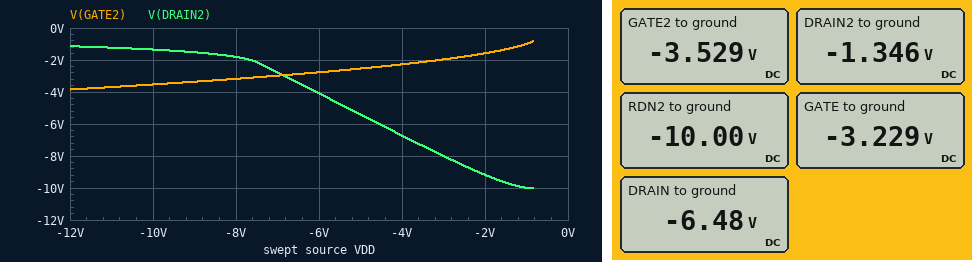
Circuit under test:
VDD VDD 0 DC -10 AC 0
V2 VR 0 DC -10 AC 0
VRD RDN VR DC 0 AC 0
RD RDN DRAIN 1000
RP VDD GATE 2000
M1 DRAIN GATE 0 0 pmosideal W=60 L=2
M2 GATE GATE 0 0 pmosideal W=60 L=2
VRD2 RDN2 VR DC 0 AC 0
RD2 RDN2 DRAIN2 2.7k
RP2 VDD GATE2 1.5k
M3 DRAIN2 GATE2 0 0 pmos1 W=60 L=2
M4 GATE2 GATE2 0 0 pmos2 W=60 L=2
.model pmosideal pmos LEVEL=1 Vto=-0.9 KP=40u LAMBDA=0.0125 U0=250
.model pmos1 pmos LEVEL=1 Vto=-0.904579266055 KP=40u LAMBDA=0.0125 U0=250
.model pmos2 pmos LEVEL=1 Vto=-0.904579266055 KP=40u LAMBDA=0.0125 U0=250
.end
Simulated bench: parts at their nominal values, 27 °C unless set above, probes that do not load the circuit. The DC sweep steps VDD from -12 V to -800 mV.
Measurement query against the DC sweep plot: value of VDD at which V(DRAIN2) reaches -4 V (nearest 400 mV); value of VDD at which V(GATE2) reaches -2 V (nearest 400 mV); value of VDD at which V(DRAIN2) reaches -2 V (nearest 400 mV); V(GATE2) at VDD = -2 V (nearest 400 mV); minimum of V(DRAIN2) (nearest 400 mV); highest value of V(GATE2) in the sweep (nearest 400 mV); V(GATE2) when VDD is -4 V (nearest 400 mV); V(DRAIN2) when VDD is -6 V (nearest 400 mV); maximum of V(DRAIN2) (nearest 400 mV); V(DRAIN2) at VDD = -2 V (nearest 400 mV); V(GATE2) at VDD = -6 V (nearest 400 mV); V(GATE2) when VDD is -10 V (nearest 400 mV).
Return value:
-6.0 V
-3.2 V
-7.6 V
-1.6 V
-10.0 V
-800 mV
-2.4 V
-4.0 V
-1.2 V
-9.2 V
-2.8 V
-3.6 V
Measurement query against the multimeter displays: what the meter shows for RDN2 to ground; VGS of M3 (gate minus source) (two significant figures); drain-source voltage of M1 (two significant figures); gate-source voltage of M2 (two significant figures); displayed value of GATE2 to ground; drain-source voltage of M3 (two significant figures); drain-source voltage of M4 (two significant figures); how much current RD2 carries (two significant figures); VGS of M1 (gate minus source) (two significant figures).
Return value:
-10.00 V
-3.5 V
-6.5 V
-3.2 V
-3.529 V
-1.3 V
-3.5 V
3.2 mA
-3.2 V
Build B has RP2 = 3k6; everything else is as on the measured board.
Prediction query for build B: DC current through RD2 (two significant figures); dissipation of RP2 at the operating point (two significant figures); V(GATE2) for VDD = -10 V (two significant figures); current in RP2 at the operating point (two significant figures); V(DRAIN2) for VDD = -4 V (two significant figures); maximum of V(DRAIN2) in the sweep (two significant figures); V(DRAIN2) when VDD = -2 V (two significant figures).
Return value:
2.1 mA
15 mW
-2.7 V
2.0 mA
-8.3 V
-3.2 V
-9.5 V
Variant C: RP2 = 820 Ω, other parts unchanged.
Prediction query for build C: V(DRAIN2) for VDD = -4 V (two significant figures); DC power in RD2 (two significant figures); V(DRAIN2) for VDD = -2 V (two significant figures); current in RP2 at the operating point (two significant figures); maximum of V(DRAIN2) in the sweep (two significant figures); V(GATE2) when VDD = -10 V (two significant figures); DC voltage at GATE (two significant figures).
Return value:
-5.2 V
30 mW
-8.9 V
7.0 mA
-840 mV
-4.2 V
-3.2 V
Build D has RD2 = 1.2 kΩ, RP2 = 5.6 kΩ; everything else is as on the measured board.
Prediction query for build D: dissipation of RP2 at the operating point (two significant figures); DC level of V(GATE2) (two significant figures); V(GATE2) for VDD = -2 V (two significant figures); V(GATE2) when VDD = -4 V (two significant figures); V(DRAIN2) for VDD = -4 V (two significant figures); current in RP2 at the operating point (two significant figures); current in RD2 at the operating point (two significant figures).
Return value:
10 mW
-2.4 V
-1.3 V
-1.7 V
-9.5 V
1.4 mA
1.5 mA
